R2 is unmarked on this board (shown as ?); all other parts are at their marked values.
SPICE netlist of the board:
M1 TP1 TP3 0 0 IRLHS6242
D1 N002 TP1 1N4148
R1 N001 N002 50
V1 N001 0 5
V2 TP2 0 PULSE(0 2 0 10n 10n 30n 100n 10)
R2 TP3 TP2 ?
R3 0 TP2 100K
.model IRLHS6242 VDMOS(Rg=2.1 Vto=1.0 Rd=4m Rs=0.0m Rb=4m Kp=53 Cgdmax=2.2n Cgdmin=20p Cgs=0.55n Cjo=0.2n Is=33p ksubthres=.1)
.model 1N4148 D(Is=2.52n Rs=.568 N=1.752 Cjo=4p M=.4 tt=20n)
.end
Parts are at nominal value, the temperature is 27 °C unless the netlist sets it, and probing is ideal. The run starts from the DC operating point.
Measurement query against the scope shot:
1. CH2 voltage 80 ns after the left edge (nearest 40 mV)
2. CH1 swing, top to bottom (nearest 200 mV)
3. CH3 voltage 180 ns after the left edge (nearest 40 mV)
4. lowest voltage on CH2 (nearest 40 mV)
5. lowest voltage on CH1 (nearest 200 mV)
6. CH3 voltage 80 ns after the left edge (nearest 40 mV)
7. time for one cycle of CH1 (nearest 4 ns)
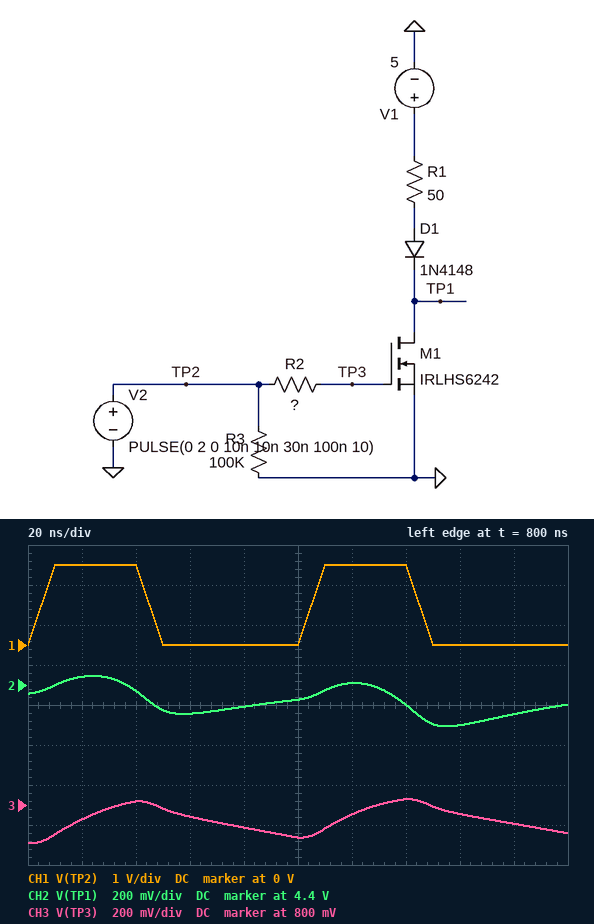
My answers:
4.28 V
2.0 V
720 mV
4.20 V
0 V
680 mV
100 ns
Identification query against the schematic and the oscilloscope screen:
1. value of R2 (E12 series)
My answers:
270 Ω
